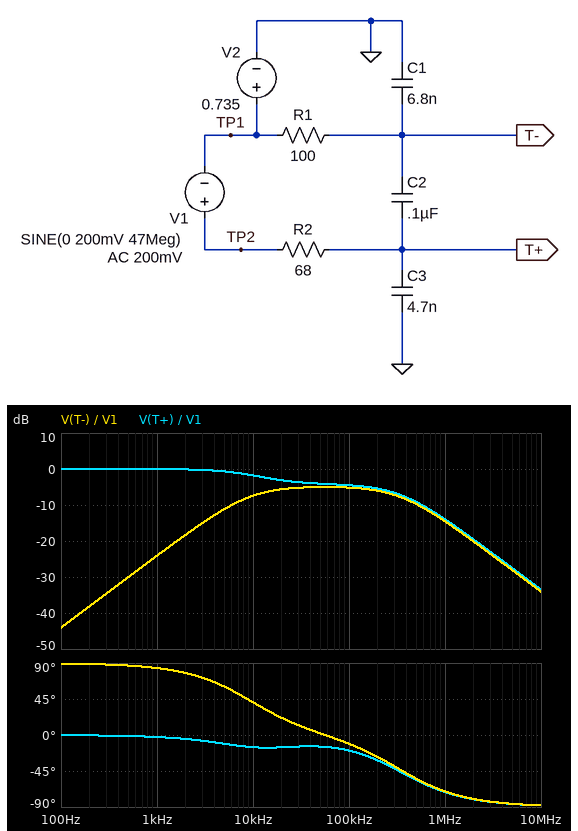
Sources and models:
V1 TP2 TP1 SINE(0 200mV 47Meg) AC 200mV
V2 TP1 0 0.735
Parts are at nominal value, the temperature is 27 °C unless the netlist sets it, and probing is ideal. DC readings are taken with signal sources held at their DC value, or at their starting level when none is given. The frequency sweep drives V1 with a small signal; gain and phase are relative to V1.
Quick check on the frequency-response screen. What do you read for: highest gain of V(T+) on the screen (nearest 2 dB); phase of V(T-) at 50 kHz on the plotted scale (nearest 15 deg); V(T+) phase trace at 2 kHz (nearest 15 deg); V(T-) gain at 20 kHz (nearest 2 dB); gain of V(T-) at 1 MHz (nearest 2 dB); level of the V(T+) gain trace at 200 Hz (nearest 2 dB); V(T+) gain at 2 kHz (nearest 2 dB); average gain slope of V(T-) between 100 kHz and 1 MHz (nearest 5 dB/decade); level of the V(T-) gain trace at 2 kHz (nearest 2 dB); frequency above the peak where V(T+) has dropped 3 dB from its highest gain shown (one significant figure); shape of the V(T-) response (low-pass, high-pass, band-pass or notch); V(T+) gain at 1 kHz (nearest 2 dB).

0 dB
0 deg
0 deg
-6 dB
-14 dB
0 dB
0 dB
-10 dB/decade
-18 dB
20 kHz
band-pass
0 dB
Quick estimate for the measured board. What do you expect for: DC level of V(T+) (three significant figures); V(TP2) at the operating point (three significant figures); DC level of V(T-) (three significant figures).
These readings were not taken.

735 mV
735 mV
735 mV
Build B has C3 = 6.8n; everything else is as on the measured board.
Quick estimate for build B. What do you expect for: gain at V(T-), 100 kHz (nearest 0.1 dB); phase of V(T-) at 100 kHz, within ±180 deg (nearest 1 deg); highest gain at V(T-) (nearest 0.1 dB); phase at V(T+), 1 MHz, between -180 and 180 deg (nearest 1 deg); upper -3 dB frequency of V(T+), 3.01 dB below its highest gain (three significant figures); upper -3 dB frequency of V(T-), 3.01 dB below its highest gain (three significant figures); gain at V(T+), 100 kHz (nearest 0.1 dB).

-5.3 dB
-14 deg
-5.1 dB
-74 deg
18.3 kHz
307 kHz
-4.7 dB
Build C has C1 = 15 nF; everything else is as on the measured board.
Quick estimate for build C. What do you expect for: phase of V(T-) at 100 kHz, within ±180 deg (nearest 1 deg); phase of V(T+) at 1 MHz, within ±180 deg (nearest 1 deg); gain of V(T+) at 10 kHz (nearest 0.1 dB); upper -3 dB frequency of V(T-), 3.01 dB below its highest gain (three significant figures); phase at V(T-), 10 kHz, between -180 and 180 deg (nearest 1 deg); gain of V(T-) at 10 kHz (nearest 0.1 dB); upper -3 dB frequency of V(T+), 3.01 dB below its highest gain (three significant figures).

-21 deg
-79 deg
-1.7 dB
222 kHz
39 deg
-7.6 dB
20.9 kHz
